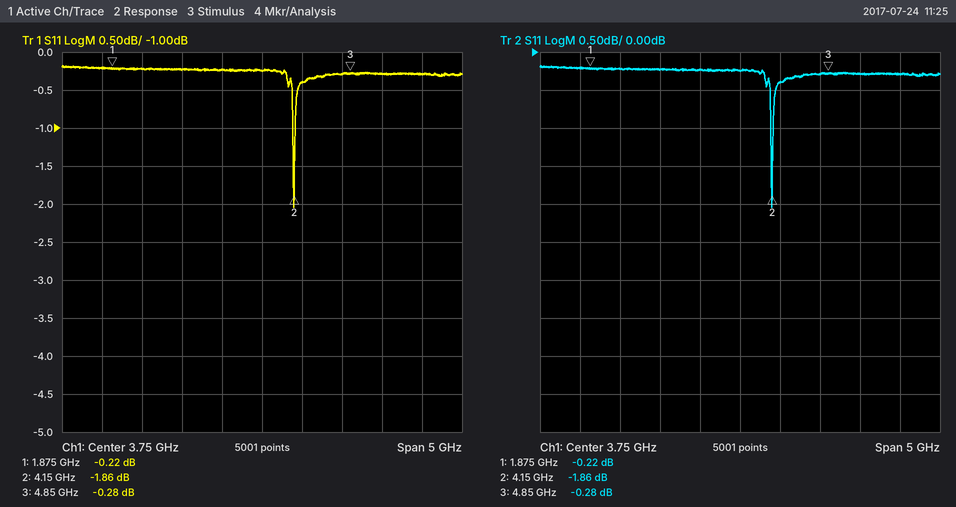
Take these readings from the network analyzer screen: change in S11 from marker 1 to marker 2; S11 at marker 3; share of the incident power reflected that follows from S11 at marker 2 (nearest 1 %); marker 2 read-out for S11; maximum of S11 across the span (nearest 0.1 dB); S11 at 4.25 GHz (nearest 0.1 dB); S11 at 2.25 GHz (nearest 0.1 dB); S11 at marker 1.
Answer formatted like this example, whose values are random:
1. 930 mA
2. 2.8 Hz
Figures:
1. -1.64 dB
2. -0.28 dB
3. 65 %
4. -1.86 dB
5. -0.2 dB
6. -0.4 dB
7. -0.2 dB
8. -0.22 dB
